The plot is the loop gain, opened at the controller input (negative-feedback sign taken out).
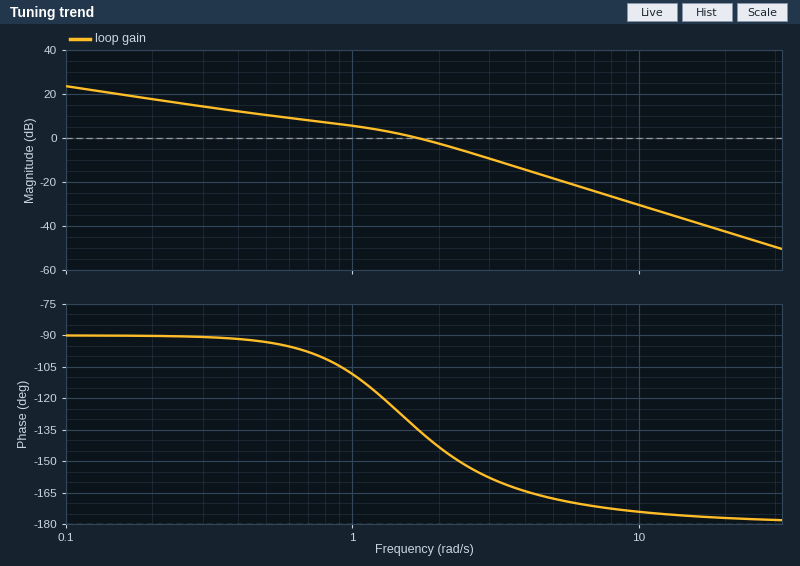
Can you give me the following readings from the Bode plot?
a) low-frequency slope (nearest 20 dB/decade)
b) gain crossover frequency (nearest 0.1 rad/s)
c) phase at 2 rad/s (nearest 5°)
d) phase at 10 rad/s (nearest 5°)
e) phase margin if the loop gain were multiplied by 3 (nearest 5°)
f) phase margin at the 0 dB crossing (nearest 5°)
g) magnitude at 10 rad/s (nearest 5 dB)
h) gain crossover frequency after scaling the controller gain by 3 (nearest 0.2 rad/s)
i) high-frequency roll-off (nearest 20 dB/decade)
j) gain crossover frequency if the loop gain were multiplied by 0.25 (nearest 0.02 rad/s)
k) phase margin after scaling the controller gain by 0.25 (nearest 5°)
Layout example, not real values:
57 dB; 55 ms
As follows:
-20 dB/decade; 1.7 rad/s; -145°; -175°; 20°; 45°; -30 dB; 3.0 rad/s; -40 dB/decade; 0.40 rad/s; 90°
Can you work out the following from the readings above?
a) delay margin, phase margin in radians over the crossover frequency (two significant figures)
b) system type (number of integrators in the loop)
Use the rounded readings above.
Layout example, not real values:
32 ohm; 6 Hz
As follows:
0.46 s; 1
